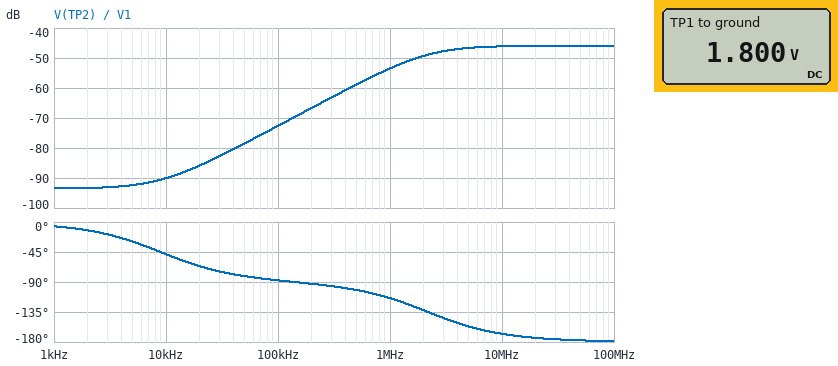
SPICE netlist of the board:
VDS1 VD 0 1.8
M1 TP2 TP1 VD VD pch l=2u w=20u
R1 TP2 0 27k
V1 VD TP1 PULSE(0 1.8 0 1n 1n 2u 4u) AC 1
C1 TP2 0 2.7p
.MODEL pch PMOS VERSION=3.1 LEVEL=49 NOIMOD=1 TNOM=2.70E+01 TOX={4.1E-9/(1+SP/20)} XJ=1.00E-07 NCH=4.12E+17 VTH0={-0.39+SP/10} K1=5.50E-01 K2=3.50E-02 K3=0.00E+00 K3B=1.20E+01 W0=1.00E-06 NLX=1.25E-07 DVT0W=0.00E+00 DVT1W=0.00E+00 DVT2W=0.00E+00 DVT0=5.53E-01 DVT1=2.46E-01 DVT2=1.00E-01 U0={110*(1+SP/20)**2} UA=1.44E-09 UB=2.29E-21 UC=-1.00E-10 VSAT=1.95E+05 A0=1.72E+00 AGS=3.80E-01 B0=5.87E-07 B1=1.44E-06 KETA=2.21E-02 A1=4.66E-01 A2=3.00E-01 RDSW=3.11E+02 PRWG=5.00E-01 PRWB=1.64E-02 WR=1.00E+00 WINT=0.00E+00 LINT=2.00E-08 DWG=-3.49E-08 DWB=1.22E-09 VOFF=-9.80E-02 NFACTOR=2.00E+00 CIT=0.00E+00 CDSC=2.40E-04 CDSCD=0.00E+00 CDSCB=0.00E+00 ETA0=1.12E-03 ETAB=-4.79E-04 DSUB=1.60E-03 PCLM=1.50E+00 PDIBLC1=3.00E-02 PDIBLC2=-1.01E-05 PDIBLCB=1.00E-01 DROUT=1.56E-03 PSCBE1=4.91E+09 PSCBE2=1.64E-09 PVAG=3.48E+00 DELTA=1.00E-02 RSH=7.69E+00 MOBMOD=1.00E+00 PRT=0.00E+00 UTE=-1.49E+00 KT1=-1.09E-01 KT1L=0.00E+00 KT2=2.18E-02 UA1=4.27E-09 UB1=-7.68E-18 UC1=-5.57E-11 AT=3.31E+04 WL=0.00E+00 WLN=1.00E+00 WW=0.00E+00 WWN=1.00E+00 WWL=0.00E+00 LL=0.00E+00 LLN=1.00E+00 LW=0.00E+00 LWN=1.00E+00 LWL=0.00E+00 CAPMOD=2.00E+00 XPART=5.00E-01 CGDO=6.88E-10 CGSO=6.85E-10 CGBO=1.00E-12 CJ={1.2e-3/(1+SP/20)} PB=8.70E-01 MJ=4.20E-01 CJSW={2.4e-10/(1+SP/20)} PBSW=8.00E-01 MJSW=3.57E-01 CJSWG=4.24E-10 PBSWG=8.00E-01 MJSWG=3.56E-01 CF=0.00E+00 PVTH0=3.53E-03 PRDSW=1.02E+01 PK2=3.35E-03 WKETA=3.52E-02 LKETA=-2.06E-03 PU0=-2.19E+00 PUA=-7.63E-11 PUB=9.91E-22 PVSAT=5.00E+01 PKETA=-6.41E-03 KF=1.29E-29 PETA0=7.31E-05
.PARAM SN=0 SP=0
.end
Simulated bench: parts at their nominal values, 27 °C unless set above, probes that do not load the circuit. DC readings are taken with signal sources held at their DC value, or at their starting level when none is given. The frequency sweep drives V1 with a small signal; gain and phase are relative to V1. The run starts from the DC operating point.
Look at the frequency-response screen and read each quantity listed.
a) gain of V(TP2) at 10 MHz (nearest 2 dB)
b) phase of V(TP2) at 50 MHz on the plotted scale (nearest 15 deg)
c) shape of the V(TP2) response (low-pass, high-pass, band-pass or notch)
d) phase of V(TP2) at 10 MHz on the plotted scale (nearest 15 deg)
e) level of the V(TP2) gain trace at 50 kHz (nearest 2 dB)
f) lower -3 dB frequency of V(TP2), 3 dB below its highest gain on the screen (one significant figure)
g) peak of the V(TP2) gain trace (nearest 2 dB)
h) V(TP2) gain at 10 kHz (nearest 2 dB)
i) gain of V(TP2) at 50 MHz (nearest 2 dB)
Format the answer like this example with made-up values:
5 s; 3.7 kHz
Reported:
-46 dB; -180 deg; high-pass; -165 deg; -78 dB; 2 MHz; -46 dB; -90 dB; -46 dB
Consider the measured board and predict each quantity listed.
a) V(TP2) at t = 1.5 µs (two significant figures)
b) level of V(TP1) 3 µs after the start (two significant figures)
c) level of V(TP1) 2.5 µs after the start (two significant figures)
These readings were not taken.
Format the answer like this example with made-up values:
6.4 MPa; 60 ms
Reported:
1.7 V; 1.8 V; 1.8 V
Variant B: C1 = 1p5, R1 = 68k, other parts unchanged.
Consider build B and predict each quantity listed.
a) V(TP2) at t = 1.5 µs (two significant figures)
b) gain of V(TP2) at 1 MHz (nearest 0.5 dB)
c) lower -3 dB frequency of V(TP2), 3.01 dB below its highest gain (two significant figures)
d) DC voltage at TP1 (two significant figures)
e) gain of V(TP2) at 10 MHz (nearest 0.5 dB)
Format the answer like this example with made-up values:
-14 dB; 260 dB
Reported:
1.8 V; -46.0 dB; 1.5 MHz; 1.8 V; -41.0 dB
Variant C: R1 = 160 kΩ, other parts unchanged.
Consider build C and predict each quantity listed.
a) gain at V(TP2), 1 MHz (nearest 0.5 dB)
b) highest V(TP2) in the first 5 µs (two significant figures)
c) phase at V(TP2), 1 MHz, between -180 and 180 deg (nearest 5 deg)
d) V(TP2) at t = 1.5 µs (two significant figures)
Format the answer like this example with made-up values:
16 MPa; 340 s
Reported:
-46.5 dB; 1.9 V; -160 deg; 1.8 V
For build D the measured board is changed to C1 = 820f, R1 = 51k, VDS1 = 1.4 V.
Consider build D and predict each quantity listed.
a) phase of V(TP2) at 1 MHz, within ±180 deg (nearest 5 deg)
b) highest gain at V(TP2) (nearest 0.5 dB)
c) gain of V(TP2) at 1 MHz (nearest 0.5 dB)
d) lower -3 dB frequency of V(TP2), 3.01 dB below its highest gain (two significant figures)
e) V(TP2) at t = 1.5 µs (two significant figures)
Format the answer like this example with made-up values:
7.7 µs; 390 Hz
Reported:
-105 deg; -35.5 dB; -47.5 dB; 3.7 MHz; 1.4 V
